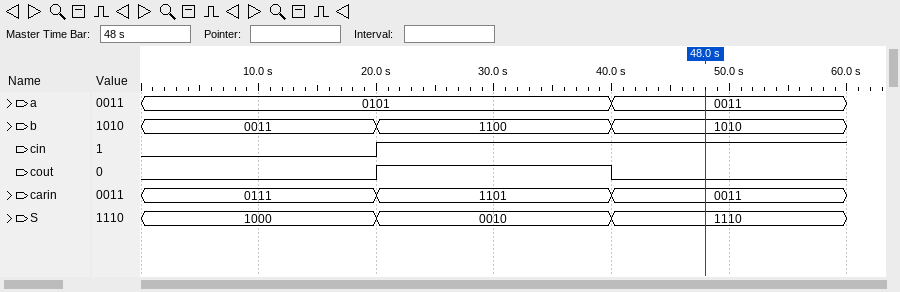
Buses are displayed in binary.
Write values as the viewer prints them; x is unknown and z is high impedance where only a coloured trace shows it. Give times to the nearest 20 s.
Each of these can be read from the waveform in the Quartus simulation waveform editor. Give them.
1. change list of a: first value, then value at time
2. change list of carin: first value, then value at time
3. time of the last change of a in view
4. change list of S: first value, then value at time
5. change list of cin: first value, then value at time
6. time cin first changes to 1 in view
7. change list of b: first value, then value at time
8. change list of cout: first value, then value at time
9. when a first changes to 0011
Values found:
0101, 0011 at 40 s
0111, 1101 at 20 s, 0011 at 40 s
40 s
1000, 0010 at 20 s, 1110 at 40 s
0, 1 at 20 s
20 s
0011, 1100 at 20 s, 1010 at 40 s
0, 1 at 20 s, 0 at 40 s
40 s
